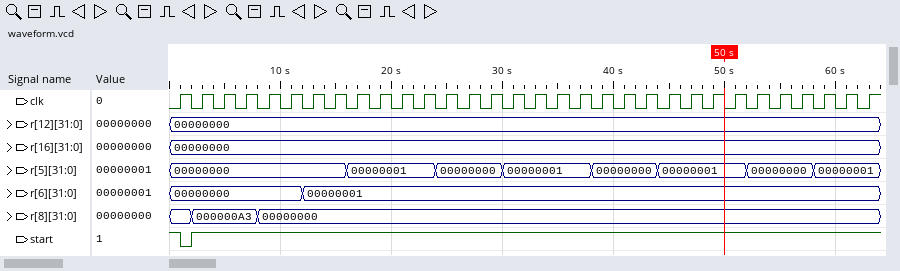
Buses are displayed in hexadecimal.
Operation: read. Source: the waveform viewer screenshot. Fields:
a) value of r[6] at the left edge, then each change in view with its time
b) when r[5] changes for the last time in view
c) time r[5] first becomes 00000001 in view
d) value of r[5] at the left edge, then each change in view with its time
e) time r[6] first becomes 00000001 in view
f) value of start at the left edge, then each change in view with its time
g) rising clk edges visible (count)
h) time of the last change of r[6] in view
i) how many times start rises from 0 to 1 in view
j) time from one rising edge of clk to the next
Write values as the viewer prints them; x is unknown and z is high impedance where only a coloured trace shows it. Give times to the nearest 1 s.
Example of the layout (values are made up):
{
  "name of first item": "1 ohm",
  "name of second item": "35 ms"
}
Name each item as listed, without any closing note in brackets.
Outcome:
{
  "value of r[6] at the left edge, then each change in view with its time": "00000000, 00000001 at 12 s",
  "when r[5] changes for the last time in view": "58 s",
  "time r[5] first becomes 00000001 in view": "16 s",
  "value of r[5] at the left edge, then each change in view with its time": "00000000, 00000001 at 16 s, 00000000 at 24 s, 00000001 at 30 s, 00000000 at 38 s, 00000001 at 44 s, 00000000 at 52 s, 00000001 at 58 s",
  "time r[6] first becomes 00000001 in view": "12 s",
  "value of start at the left edge, then each change in view with its time": "1, 0 at 1 s, 1 at 2 s",
  "rising clk edges visible": "32",
  "time of the last change of r[6] in view": "12 s",
  "how many times start rises from 0 to 1 in view": "1",
  "time from one rising edge of clk to the next": "2 s"
}
